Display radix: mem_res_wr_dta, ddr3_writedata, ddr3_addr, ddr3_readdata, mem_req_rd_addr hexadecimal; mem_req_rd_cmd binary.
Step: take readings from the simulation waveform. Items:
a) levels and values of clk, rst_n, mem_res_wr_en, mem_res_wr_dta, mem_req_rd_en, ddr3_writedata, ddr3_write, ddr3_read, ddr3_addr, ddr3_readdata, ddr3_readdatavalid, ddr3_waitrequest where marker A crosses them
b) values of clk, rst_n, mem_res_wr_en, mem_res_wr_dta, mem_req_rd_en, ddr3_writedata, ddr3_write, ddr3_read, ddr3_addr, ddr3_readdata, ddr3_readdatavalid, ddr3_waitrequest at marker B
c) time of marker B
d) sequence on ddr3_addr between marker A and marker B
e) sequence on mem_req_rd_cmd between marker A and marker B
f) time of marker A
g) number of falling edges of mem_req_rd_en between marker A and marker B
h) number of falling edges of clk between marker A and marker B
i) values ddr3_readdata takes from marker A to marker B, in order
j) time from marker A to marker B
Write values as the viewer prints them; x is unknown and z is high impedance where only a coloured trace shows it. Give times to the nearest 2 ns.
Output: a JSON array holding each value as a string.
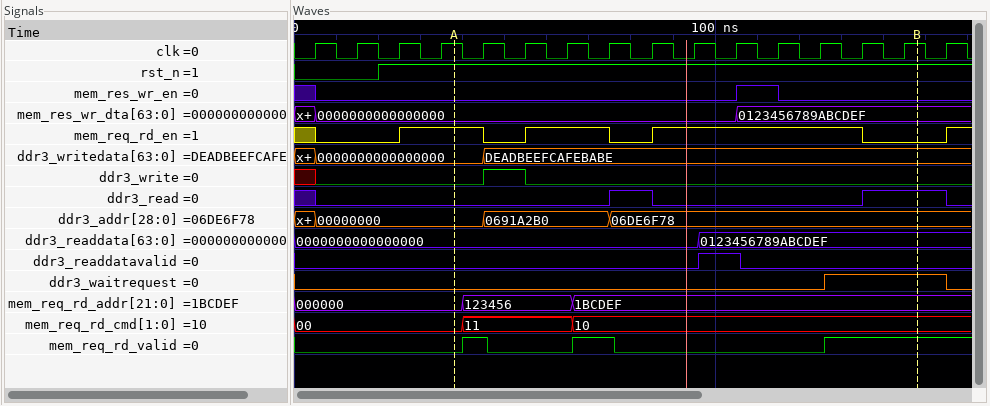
["clk=1, rst_n=1, mem_res_wr_en=0, mem_res_wr_dta=0000000000000000, mem_req_rd_en=1, ddr3_writedata=0000000000000000, ddr3_write=0, ddr3_read=0, ddr3_addr=00000000, ddr3_readdata=0000000000000000, ddr3_readdatavalid=0, ddr3_waitrequest=0", "clk=1, rst_n=1, mem_res_wr_en=0, mem_res_wr_dta=0123456789ABCDEF, mem_req_rd_en=0, ddr3_writedata=DEADBEEFCAFEBABE, ddr3_write=0, ddr3_read=1, ddr3_addr=06DE6F78, ddr3_readdata=0123456789ABCDEF, ddr3_readdatavalid=0, ddr3_waitrequest=1", "148 ns", "00000000, 0691A2B0, 06DE6F78", "00, 11, 10", "38 ns", "3", "11", "0000000000000000, 0123456789ABCDEF", "110 ns"]
